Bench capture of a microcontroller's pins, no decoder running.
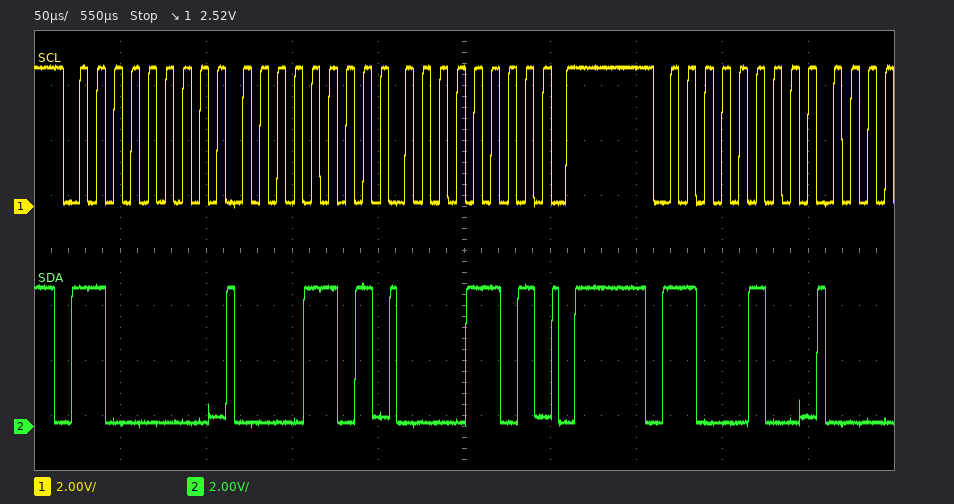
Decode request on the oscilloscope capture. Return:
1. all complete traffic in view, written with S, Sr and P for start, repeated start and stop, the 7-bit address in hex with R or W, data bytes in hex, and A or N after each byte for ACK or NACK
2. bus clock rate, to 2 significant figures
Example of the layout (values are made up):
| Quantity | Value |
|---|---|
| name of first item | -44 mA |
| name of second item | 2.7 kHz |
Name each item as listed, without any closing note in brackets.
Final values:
| Quantity | Value |
|---|---|
| all complete traffic in view, written with S, Sr and P for start, repeated start and stop, the 7-bit address in hex with R or W, data bytes in hex, and A or N after each byte for ACK or NACK | S 60W A 0D A 0D A P S 62W A |
| bus clock rate, to 2 significant figures | 100 kHz |
